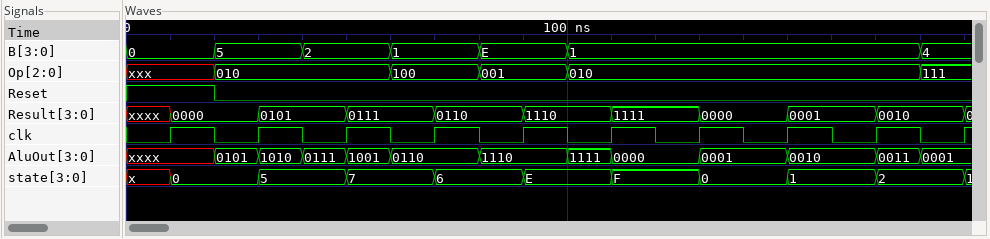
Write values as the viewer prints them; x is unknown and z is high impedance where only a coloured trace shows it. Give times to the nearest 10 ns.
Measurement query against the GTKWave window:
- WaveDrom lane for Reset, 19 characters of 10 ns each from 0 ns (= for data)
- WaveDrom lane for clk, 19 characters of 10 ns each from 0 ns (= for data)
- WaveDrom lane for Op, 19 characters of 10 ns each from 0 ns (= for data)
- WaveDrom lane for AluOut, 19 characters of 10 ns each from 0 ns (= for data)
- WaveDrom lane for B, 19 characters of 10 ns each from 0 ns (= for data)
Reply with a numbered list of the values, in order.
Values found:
1. {name: 'Reset', wave: '1.0................'}
2. {name: 'clk', wave: '0101010101010101010'}
3. {name: 'Op', wave: 'x.=...=.=.=.......=', data: '010 100 001 010 111'}
4. {name: 'AluOut', wave: 'x.=====.=.==.=.=.==', data: '0101 1010 0111 1001 0110 1110 1111 0000 0001 0010 0011 0001'}
5. {name: 'B', wave: '=.=.=.=.=.=.......=', data: '0 5 2 1 E 1 4'}
